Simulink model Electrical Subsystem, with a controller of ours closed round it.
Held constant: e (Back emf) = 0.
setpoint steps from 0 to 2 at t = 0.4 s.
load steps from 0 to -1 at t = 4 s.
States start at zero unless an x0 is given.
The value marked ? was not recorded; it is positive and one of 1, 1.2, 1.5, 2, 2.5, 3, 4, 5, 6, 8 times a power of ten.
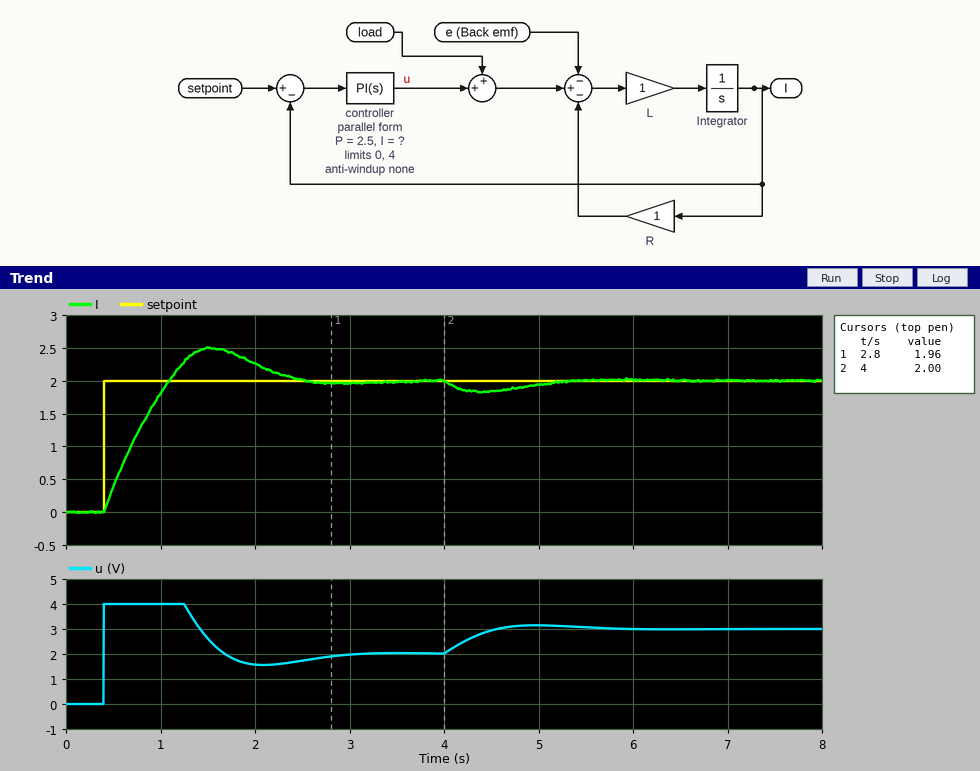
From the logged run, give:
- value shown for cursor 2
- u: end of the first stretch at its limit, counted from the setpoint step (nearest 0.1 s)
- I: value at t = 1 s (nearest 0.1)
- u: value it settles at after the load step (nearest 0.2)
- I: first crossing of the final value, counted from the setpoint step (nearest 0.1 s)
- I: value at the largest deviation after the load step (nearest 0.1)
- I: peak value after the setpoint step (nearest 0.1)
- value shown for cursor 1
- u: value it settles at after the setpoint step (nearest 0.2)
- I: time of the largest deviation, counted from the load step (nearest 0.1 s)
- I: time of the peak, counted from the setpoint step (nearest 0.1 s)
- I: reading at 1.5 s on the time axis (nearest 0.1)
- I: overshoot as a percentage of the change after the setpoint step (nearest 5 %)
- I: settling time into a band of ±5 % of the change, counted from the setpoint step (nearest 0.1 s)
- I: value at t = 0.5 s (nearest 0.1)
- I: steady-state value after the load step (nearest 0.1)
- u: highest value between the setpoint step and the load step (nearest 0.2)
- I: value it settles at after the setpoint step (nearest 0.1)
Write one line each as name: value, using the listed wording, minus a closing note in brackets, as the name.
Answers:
value shown for cursor 2: 2.00
u: end of the first stretch at its limit, counted from the setpoint step: 0.9 s
I: value at t = 1 s: 1.8
u: value it settles at after the load step: 3.0
I: first crossing of the final value, counted from the setpoint step: 0.7 s
I: value at the largest deviation after the load step: 1.8
I: peak value after the setpoint step: 2.5
value shown for cursor 1: 1.96
u: value it settles at after the setpoint step: 2.0
I: time of the largest deviation, counted from the load step: 0.4 s
I: time of the peak, counted from the setpoint step: 1.1 s
I: reading at 1.5 s on the time axis: 2.5
I: overshoot as a percentage of the change after the setpoint step: 25 %
I: settling time into a band of ±5 % of the change, counted from the setpoint step: 1.9 s
I: value at t = 0.5 s: 0.4
I: steady-state value after the load step: 2.0
u: highest value between the setpoint step and the load step: 4.0
I: value it settles at after the setpoint step: 2.0
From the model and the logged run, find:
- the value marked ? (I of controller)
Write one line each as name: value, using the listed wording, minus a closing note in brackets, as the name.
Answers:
the value marked ?: 8
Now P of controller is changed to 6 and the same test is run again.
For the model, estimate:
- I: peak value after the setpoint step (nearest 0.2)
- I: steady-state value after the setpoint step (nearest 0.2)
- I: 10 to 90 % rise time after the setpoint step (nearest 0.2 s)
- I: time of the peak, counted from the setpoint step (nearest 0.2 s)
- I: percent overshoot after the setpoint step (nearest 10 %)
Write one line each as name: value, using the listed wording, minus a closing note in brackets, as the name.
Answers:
I: peak value after the setpoint step: 2.4
I: steady-state value after the setpoint step: 2.0
I: 10 to 90 % rise time after the setpoint step: 0.6 s
I: time of the peak, counted from the setpoint step: 1.0 s
I: percent overshoot after the setpoint step: 20 %
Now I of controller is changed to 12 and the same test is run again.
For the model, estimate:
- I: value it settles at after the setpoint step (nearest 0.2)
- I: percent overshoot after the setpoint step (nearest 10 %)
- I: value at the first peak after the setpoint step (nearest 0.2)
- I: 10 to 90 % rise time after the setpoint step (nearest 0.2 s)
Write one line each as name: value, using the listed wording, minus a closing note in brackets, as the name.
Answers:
I: value it settles at after the setpoint step: 2.0
I: percent overshoot after the setpoint step: 40 %
I: value at the first peak after the setpoint step: 2.8
I: 10 to 90 % rise time after the setpoint step: 0.6 s
